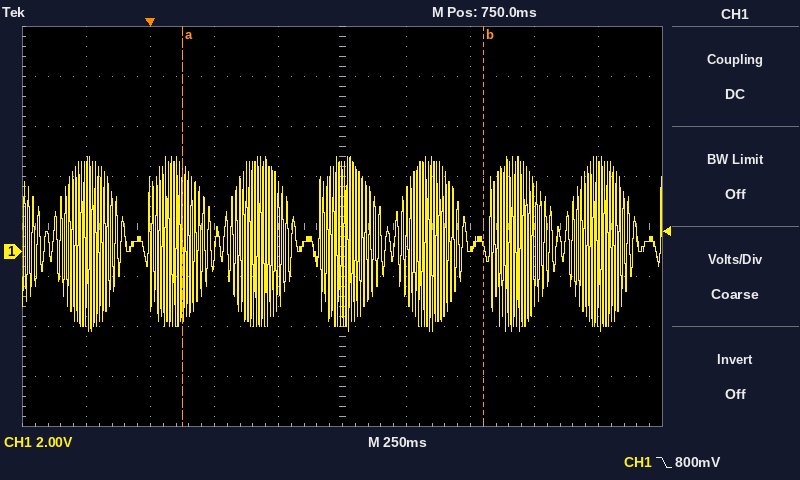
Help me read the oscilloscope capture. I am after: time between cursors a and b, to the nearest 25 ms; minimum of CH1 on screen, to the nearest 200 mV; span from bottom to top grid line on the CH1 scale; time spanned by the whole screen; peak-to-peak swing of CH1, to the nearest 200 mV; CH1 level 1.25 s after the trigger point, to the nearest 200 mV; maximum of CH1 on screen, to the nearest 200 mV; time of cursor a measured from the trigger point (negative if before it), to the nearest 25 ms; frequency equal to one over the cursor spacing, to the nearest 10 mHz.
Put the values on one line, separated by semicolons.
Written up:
1.175 s; -3.2 V; 16 V; 2.5 s; 7.0 V; 200 mV; 3.8 V; +125 ms; 850 mHz
